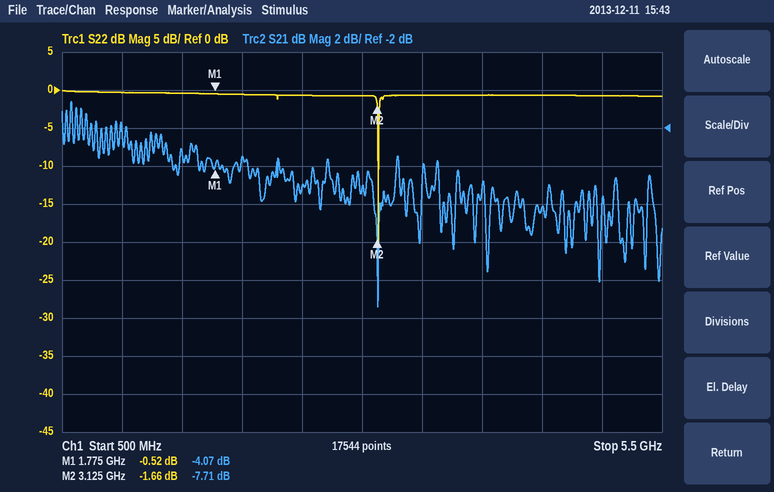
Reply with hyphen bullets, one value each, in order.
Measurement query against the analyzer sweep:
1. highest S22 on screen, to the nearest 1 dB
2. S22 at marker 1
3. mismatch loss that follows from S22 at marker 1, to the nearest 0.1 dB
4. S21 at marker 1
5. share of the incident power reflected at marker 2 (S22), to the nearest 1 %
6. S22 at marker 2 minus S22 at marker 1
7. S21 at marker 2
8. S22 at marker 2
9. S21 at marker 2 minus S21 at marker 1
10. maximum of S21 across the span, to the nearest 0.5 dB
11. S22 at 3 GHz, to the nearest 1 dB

- 0 dB
- -0.52 dB
- 9.5 dB
- -4.07 dB
- 68 %
- -1.14 dB
- -7.71 dB
- -1.66 dB
- -3.64 dB
- -0.5 dB
- -1 dB
